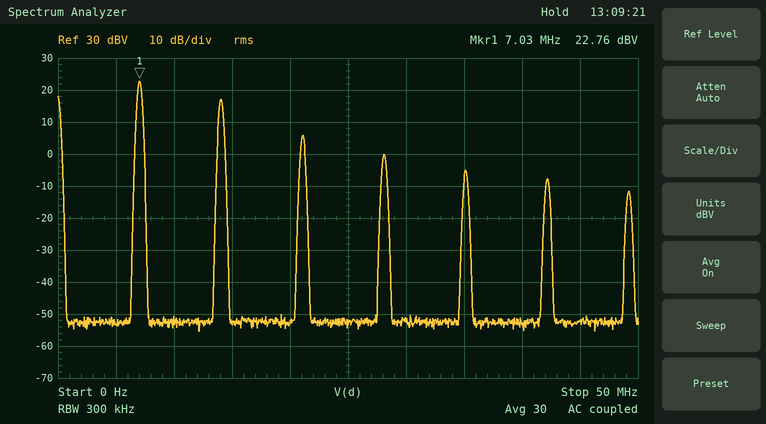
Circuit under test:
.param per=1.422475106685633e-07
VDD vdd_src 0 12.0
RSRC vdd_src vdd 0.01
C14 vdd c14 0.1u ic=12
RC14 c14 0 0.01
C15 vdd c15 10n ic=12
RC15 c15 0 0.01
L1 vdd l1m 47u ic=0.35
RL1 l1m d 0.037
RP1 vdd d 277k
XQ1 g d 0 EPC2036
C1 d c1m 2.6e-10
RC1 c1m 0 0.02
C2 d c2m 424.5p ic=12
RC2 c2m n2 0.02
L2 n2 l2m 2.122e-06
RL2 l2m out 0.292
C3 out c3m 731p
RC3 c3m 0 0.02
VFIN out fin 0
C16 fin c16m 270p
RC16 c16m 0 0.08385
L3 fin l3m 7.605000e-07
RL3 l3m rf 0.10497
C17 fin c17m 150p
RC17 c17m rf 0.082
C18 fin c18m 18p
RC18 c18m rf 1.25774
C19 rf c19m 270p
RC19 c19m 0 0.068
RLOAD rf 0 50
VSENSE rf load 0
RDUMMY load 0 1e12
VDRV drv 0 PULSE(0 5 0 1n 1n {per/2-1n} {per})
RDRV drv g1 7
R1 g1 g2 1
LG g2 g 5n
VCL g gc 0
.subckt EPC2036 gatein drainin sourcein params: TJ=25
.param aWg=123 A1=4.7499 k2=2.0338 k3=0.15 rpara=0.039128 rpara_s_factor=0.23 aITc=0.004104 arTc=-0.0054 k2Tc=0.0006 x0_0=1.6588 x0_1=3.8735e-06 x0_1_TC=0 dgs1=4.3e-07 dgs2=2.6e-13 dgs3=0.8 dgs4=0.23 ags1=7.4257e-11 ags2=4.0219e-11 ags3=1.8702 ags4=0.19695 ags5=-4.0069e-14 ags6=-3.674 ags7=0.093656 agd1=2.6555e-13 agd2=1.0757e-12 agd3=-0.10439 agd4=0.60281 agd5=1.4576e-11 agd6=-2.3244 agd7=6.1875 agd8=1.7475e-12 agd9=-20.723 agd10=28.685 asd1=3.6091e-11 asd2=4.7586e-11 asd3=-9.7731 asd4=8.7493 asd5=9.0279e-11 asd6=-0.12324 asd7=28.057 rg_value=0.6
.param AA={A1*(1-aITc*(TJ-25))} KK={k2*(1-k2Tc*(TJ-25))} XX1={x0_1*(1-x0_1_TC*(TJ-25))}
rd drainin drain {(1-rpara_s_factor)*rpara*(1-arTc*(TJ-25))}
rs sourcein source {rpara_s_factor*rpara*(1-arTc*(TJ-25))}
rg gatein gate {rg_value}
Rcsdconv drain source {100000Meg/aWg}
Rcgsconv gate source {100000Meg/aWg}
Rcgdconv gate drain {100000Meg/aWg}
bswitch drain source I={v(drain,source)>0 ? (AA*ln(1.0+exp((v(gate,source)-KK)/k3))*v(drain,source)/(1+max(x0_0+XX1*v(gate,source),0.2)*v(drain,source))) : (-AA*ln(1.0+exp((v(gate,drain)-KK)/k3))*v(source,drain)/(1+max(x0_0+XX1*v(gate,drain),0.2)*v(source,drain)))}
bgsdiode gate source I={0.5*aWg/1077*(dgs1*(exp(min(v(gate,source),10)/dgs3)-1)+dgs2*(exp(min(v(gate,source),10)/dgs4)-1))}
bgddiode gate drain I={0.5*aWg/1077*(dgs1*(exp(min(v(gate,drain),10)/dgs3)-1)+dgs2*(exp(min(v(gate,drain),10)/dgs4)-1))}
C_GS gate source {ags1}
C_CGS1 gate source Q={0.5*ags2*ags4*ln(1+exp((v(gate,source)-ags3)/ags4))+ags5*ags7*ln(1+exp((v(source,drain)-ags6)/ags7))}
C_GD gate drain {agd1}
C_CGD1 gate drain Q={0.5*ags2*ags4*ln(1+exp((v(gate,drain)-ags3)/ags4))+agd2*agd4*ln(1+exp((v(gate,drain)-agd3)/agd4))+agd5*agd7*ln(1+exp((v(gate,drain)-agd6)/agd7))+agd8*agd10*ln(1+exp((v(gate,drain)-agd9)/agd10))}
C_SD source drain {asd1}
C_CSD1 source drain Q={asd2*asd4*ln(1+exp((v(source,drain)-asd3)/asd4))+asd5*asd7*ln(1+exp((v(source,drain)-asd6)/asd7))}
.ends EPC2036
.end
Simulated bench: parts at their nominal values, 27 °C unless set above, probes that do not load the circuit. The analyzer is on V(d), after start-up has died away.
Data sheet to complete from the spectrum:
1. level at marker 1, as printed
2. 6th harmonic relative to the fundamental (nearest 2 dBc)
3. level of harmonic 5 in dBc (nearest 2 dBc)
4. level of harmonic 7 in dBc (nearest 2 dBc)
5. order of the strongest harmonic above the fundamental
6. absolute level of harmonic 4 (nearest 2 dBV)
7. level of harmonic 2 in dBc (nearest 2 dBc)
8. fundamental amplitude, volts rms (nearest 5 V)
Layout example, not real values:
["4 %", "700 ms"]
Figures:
["22.76 dBV", "-30 dBc", "-28 dBc", "-34 dBc", "2", "0 dBV", "-6 dBc", "15 V"]
